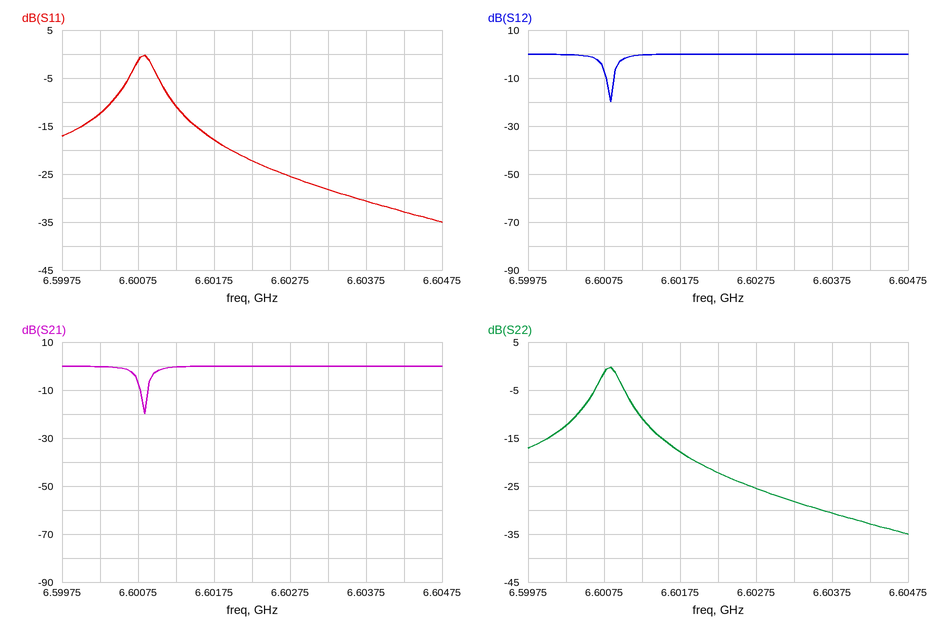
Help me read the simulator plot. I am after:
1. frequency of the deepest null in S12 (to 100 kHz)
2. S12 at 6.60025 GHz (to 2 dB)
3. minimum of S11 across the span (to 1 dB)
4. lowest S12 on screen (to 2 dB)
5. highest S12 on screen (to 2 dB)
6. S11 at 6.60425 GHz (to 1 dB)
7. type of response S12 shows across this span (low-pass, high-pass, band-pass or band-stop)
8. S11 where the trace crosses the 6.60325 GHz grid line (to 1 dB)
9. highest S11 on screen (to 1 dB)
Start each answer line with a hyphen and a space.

- 6.6008 GHz
- 0 dB
- -35 dB
- -20 dB
- 0 dB
- -33 dB
- band-stop
- -28 dB
- 0 dB
